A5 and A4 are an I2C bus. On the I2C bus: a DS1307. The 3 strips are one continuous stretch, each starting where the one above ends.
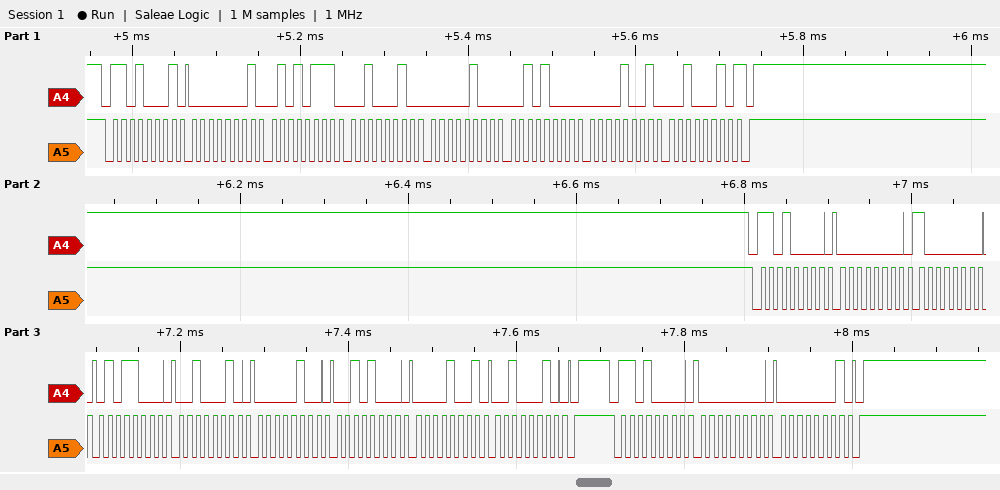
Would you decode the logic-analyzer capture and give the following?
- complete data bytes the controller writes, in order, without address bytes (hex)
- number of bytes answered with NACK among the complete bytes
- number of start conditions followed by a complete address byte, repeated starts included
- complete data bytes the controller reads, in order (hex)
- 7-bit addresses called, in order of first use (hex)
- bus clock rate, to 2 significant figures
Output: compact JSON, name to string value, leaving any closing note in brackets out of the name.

{"complete data bytes the controller writes, in order, without address bytes": "00 80 58 22 04 28 09 22 00 01", "number of bytes answered with NACK among the complete bytes": "1", "number of start conditions followed by a complete address byte, repeated starts included": "3", "complete data bytes the controller reads, in order": "01 57 22 04 28 09 22", "7-bit addresses called, in order of first use": "0x68", "bus clock rate, to 2 significant figures": "100 kHz"}
